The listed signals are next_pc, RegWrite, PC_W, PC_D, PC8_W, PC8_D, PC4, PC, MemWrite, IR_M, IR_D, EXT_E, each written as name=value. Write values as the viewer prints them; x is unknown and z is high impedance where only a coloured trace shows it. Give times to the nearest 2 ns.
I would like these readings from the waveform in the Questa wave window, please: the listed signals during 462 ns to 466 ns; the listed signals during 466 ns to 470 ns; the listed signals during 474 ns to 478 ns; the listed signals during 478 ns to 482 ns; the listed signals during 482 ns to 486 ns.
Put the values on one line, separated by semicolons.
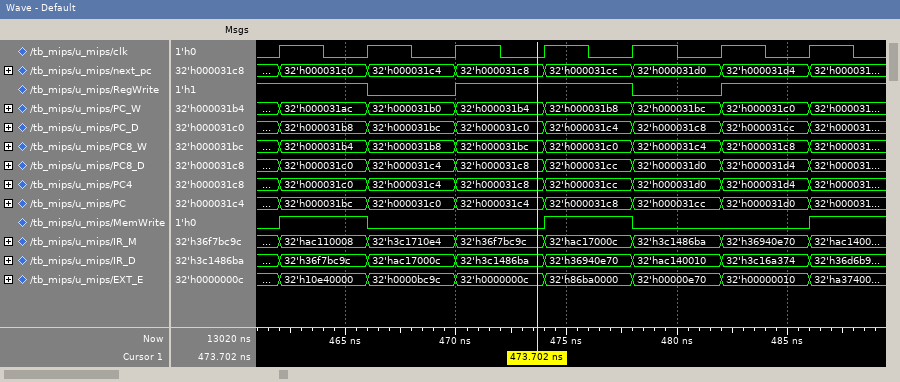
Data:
next_pc=32'h000031c0, RegWrite=1, PC_W=32'h000031ac, PC_D=32'h000031b8, PC8_W=32'h000031b4, PC8_D=32'h000031c0, PC4=32'h000031c0, PC=32'h000031bc, MemWrite=1, IR_M=32'hac110008, IR_D=32'h36f7bc9c, EXT_E=32'h10e40000; next_pc=32'h000031c4, RegWrite=0, PC_W=32'h000031b0, PC_D=32'h000031bc, PC8_W=32'h000031b8, PC8_D=32'h000031c4, PC4=32'h000031c4, PC=32'h000031c0, MemWrite=0, IR_M=32'h3c1710e4, IR_D=32'hac17000c, EXT_E=32'h0000bc9c; next_pc=32'h000031cc, RegWrite=1, PC_W=32'h000031b8, PC_D=32'h000031c4, PC8_W=32'h000031c0, PC8_D=32'h000031cc, PC4=32'h000031cc, PC=32'h000031c8, MemWrite=1, IR_M=32'hac17000c, IR_D=32'h36940e70, EXT_E=32'h86ba0000; next_pc=32'h000031d0, RegWrite=0, PC_W=32'h000031bc, PC_D=32'h000031c8, PC8_W=32'h000031c4, PC8_D=32'h000031d0, PC4=32'h000031d0, PC=32'h000031cc, MemWrite=0, IR_M=32'h3c1486ba, IR_D=32'hac140010, EXT_E=32'h00000e70; next_pc=32'h000031d4, RegWrite=1, PC_W=32'h000031c0, PC_D=32'h000031cc, PC8_W=32'h000031c8, PC8_D=32'h000031d4, PC4=32'h000031d4, PC=32'h000031d0, MemWrite=0, IR_M=32'h36940e70, IR_D=32'h3c16a374, EXT_E=32'h00000010
